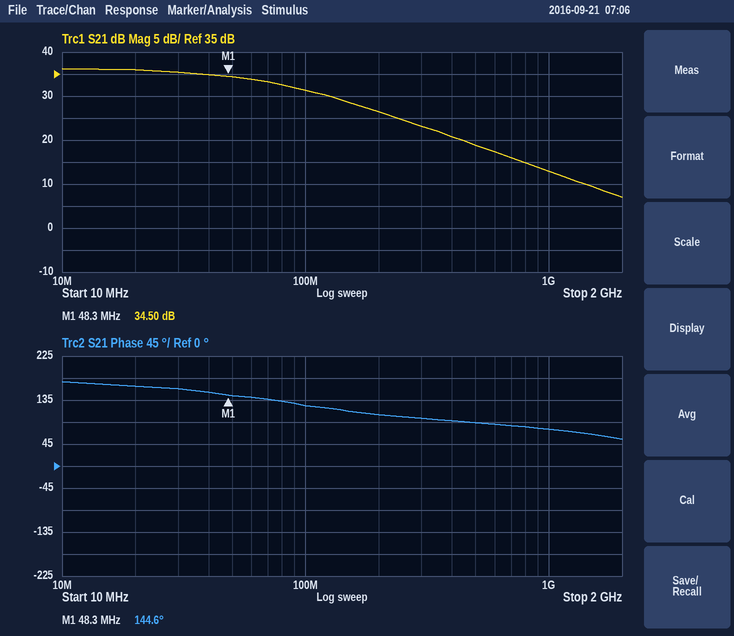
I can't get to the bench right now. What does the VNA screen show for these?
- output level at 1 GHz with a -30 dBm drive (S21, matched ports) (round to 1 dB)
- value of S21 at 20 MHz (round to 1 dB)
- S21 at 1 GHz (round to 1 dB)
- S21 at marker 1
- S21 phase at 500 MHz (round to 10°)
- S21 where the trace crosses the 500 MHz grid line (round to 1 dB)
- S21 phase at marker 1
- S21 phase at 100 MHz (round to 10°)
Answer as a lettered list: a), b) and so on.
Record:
a) -17 dBm
b) 36 dB
c) 13 dB
d) 34.50 dB
e) 90°
f) 19 dB
g) 144.6°
h) 120°
